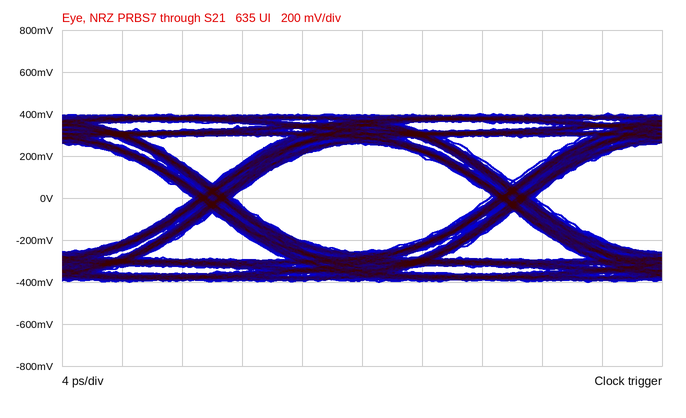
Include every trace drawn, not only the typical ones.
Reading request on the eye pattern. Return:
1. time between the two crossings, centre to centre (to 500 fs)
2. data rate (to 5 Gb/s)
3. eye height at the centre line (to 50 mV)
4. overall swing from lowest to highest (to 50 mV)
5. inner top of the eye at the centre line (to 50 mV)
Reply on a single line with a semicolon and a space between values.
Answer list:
20.0 ps; 50 Gb/s; 500 mV; 800 mV; 250 mV
